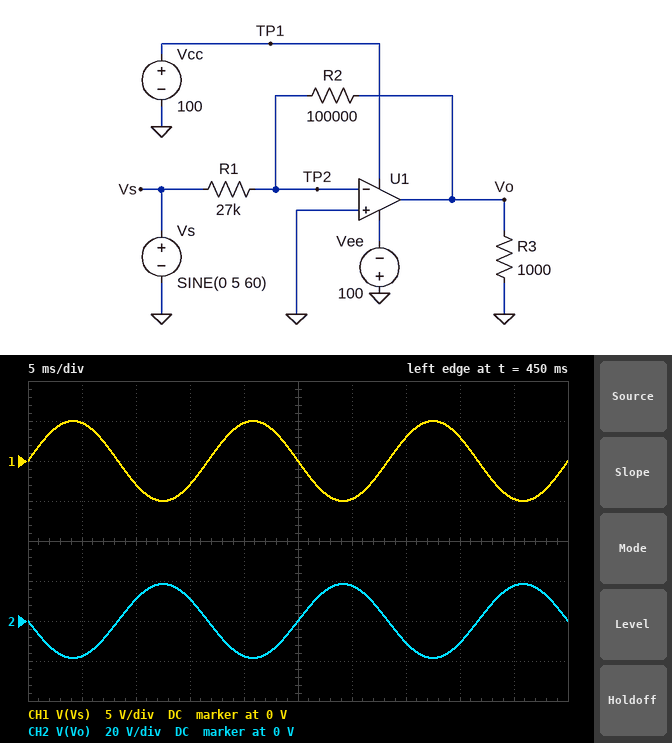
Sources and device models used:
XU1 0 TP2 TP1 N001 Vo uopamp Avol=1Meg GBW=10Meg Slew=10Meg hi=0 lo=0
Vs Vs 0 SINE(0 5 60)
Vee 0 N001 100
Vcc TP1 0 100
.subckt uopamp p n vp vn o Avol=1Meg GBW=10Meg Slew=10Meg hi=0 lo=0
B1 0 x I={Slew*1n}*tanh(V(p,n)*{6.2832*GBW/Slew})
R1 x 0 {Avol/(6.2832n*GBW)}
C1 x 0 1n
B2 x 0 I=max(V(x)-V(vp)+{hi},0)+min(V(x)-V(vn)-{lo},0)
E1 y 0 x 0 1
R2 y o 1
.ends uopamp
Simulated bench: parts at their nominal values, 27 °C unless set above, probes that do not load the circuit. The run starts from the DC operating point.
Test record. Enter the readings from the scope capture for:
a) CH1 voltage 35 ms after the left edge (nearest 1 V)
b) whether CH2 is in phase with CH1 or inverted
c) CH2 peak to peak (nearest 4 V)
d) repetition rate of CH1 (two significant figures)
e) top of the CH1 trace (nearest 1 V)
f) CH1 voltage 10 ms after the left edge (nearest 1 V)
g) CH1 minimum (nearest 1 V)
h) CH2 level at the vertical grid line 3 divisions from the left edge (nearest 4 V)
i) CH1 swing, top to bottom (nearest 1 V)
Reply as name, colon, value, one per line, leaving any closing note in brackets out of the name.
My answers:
CH1 voltage 35 ms after the left edge: 3 V
whether CH2 is in phase with CH1 or inverted: inverted
CH2 peak to peak: 36 V
repetition rate of CH1: 60 Hz
top of the CH1 trace: 5 V
CH1 voltage 10 ms after the left edge: -3 V
CH1 minimum: -5 V
CH2 level at the vertical grid line 3 divisions from the left edge: 12 V
CH1 swing, top to bottom: 10 V
